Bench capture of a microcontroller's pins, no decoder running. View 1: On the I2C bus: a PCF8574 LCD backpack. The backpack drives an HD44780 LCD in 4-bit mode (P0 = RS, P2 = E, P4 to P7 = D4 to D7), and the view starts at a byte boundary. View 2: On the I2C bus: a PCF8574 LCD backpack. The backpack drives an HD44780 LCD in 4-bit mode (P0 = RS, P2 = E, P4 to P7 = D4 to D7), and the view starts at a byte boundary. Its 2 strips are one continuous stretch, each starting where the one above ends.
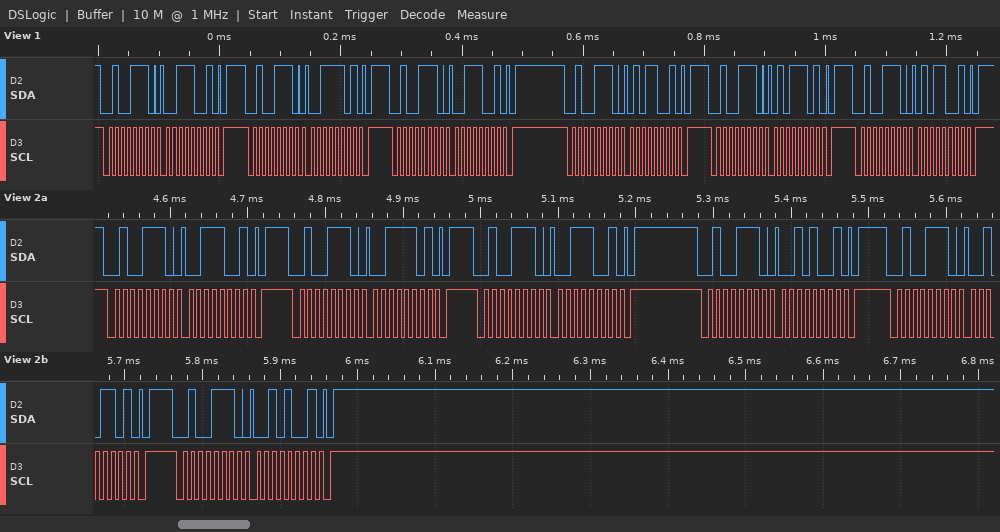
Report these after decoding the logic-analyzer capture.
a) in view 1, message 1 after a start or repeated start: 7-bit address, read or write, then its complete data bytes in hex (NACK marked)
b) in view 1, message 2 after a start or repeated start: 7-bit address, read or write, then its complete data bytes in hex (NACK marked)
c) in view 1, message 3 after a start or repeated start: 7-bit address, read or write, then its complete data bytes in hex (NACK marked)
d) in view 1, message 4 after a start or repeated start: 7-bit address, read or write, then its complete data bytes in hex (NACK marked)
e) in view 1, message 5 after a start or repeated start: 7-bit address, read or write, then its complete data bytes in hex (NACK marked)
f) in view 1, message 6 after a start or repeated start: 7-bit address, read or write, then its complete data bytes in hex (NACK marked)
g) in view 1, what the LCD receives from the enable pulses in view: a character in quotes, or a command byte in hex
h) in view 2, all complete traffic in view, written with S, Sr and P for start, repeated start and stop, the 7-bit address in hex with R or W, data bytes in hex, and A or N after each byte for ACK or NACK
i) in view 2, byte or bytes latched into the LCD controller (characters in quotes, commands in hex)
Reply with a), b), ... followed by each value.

a) 0x27 write: 39
b) 0x27 write: 3D
c) 0x27 write: 39
d) 0x27 write: 59
e) 0x27 write: 5D
f) 0x27 write: 59
g) '5'
h) S 27W A 39 A P S 27W A 3D A P S 27W A 39 A P S 27W A 29 A P S 27W A 2D A P S 27W A 29 A P
i) '2'
